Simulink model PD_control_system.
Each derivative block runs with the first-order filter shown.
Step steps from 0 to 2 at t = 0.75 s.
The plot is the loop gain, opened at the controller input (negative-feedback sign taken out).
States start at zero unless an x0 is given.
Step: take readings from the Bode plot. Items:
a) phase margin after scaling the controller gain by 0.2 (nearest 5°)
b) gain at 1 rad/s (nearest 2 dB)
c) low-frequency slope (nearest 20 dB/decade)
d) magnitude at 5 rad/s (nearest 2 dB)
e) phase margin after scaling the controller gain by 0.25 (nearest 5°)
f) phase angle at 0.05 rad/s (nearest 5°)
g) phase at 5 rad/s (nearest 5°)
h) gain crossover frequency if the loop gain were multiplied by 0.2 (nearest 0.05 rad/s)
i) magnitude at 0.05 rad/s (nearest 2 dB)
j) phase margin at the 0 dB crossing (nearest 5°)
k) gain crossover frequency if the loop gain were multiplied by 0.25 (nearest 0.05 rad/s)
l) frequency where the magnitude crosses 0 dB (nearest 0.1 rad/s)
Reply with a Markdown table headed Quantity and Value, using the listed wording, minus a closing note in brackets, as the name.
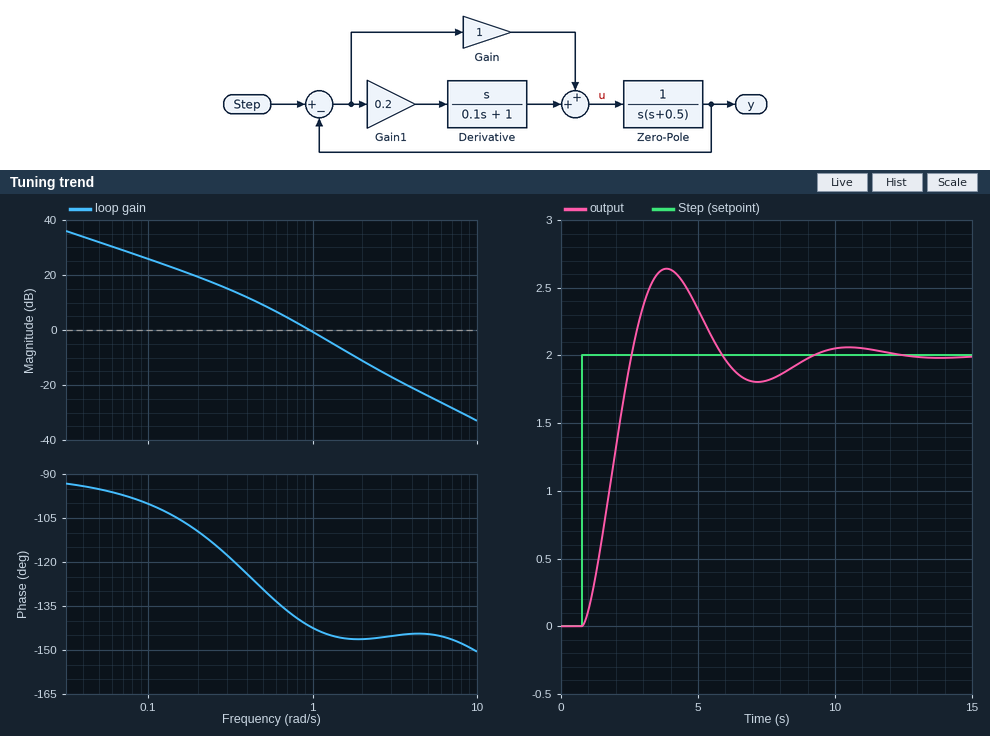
| Quantity | Value |
|---|---|
| phase margin after scaling the controller gain by 0.2 | 60° |
| gain at 1 rad/s | 0 dB |
| low-frequency slope | -20 dB/decade |
| magnitude at 5 rad/s | -24 dB |
| phase margin after scaling the controller gain by 0.25 | 55° |
| phase angle at 0.05 rad/s | -95° |
| phase at 5 rad/s | -145° |
| gain crossover frequency if the loop gain were multiplied by 0.2 | 0.35 rad/s |
| magnitude at 0.05 rad/s | 32 dB |
| phase margin at the 0 dB crossing | 40° |
| gain crossover frequency if the loop gain were multiplied by 0.25 | 0.40 rad/s |
| frequency where the magnitude crosses 0 dB | 1.0 rad/s |
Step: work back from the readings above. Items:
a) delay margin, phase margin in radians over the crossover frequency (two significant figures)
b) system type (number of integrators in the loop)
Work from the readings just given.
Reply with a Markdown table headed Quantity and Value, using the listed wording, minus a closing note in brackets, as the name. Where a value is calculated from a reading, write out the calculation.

| Quantity | Value |
|---|---|
| delay margin, phase margin in radians over the crossover frequency | 40 × π / 180 / 1 = 0.70 s |
| system type | 1 |
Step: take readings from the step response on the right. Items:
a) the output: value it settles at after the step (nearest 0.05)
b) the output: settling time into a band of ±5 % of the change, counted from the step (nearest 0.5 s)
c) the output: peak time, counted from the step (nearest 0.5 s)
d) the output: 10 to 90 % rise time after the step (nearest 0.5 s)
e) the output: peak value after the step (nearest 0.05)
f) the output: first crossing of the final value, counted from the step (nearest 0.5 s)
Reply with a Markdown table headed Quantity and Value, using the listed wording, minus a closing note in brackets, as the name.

| Quantity | Value |
|---|---|
| the output: value it settles at after the step | 2.00 |
| the output: settling time into a band of ±5 % of the change, counted from the step | 7.5 s |
| the output: peak time, counted from the step | 3.0 s |
| the output: 10 to 90 % rise time after the step | 1.5 s |
| the output: peak value after the step | 2.65 |
| the output: first crossing of the final value, counted from the step | 2.0 s |
